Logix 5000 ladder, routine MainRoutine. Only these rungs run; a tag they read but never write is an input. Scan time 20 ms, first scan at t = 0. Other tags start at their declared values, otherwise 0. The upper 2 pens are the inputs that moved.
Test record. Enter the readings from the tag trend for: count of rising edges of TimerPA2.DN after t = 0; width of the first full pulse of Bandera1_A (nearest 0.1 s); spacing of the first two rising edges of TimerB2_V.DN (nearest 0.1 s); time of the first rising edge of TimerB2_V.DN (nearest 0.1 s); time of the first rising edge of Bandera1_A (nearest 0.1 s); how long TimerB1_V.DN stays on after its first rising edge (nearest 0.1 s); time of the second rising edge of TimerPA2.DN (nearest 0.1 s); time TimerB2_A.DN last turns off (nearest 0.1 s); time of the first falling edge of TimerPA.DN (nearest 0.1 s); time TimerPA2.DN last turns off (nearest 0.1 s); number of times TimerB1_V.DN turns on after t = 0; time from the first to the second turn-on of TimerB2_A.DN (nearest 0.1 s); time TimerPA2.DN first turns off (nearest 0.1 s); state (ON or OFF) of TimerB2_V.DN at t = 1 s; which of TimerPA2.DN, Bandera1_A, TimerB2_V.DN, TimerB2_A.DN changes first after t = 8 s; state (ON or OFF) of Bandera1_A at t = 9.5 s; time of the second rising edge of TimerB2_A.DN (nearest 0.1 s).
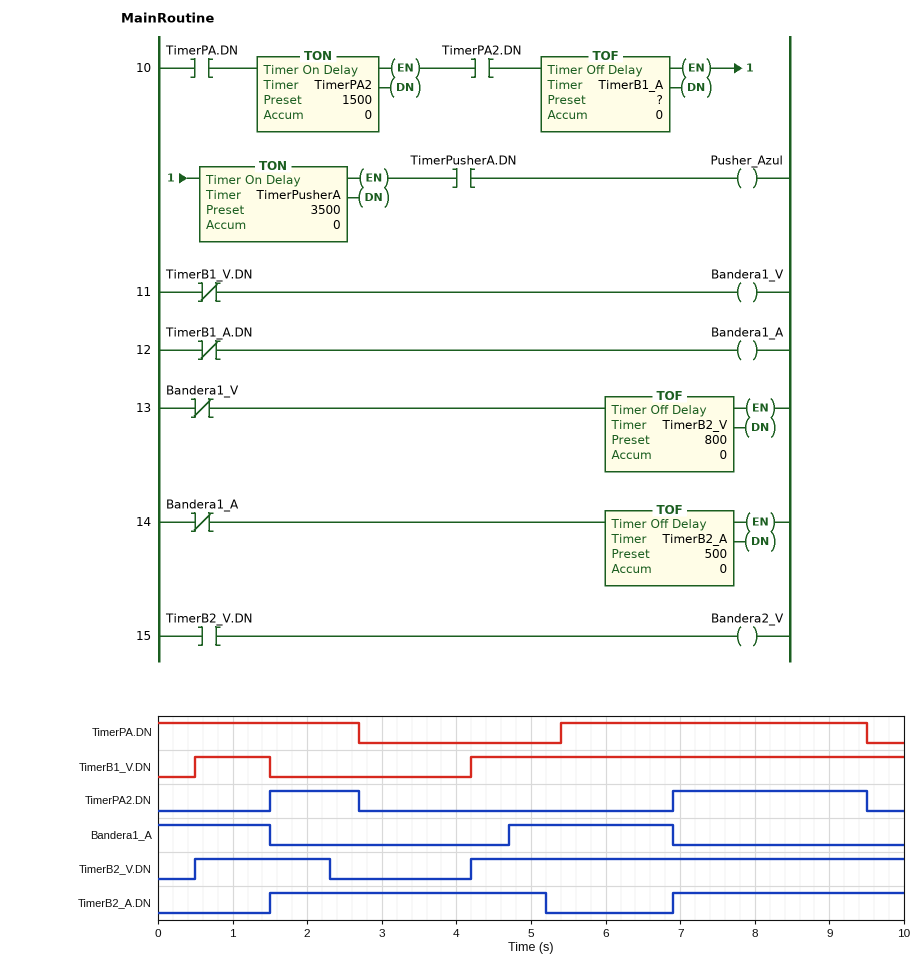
2
2.2 s
3.7 s
0.5 s
4.7 s
1.0 s
6.9 s
5.2 s
2.7 s
9.5 s
2
5.4 s
2.7 s
ON
TimerPA2.DN
OFF
6.9 s
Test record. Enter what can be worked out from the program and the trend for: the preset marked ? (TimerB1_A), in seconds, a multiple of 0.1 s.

2.0 s
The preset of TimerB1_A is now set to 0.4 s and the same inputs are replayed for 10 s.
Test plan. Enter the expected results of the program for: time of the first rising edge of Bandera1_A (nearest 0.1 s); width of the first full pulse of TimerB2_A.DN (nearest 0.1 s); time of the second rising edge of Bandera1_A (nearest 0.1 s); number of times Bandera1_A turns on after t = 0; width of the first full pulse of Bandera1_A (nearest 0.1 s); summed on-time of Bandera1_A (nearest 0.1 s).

3.1 s
2.1 s
9.9 s
2
3.8 s
5.4 s
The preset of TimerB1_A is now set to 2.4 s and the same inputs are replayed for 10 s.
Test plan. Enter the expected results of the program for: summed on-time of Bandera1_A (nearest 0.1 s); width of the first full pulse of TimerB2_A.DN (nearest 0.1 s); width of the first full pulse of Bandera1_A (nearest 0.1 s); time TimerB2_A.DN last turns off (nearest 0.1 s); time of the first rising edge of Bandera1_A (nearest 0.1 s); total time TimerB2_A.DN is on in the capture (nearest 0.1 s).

3.3 s
4.1 s
1.8 s
5.6 s
5.1 s
7.2 s
